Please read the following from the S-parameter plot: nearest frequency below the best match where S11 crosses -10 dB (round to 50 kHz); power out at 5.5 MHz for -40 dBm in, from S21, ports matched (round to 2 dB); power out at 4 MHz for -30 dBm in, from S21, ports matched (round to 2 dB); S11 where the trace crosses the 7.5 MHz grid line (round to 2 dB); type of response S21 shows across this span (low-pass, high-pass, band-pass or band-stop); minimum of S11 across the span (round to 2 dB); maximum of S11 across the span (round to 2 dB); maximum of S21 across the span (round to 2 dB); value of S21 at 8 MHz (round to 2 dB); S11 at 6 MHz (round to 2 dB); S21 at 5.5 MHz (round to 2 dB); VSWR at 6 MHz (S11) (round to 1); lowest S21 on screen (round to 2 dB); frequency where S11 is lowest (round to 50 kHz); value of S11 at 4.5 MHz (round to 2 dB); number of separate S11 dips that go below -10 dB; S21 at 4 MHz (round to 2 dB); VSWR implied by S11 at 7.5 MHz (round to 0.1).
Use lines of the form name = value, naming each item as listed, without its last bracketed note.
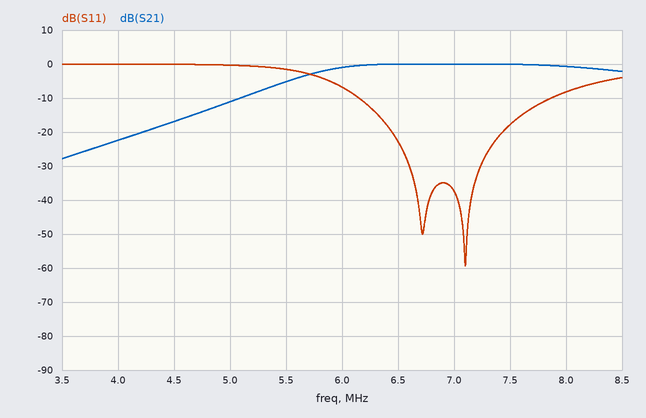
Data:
nearest frequency below the best match where S11 crosses -10 dB = 6.15 MHz
power out at 5.5 MHz for -40 dBm in, from S21, ports matched = -46 dBm
power out at 4 MHz for -30 dBm in, from S21, ports matched = -52 dBm
S11 where the trace crosses the 7.5 MHz grid line = -18 dB
type of response S21 shows across this span = high-pass
minimum of S11 across the span = -60 dB
maximum of S11 across the span = 0 dB
maximum of S21 across the span = 0 dB
value of S21 at 8 MHz = 0 dB
S11 at 6 MHz = -6 dB
S21 at 5.5 MHz = -6 dB
VSWR at 6 MHz (S11) = 3
lowest S21 on screen = -28 dB
frequency where S11 is lowest = 7.10 MHz
value of S11 at 4.5 MHz = 0 dB
number of separate S11 dips that go below -10 dB = 2
S21 at 4 MHz = -22 dB
VSWR implied by S11 at 7.5 MHz = 1.3
